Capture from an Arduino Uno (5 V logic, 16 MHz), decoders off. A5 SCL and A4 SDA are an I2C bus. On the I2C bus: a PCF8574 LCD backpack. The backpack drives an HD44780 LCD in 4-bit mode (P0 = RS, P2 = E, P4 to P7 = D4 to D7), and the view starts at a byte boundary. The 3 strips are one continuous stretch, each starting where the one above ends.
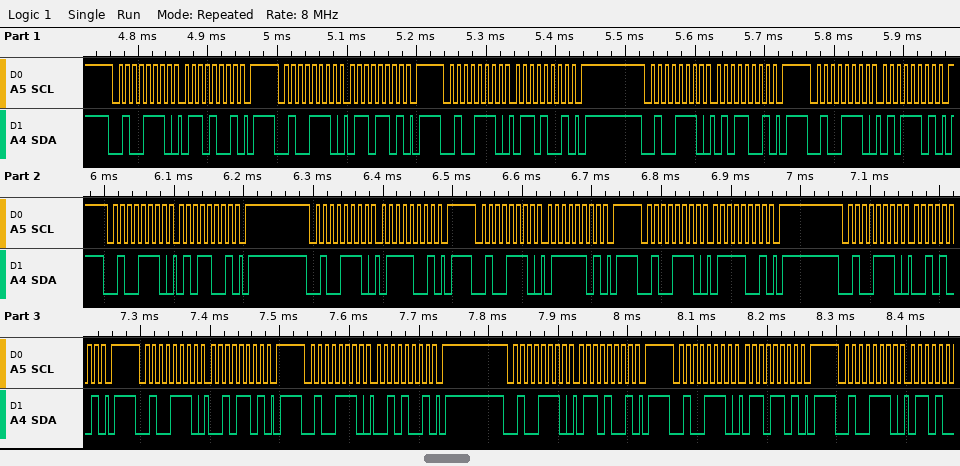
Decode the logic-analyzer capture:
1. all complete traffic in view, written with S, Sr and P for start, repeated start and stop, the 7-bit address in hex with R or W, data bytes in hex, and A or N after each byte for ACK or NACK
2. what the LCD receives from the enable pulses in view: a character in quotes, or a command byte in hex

S 27W A 69 A P S 27W A 6D A P S 27W A 69 A P S 27W A 59 A P S 27W A 5D A P S 27W A 59 A P S 27W A 79 A P S 27W A 7D A P S 27W A 79 A P S 27W A 29 A P S 27W A 2D A P S 27W A 29 A P S 27W A 69 A P S 27W A 6D A P S 27W A
'e' 'r'
